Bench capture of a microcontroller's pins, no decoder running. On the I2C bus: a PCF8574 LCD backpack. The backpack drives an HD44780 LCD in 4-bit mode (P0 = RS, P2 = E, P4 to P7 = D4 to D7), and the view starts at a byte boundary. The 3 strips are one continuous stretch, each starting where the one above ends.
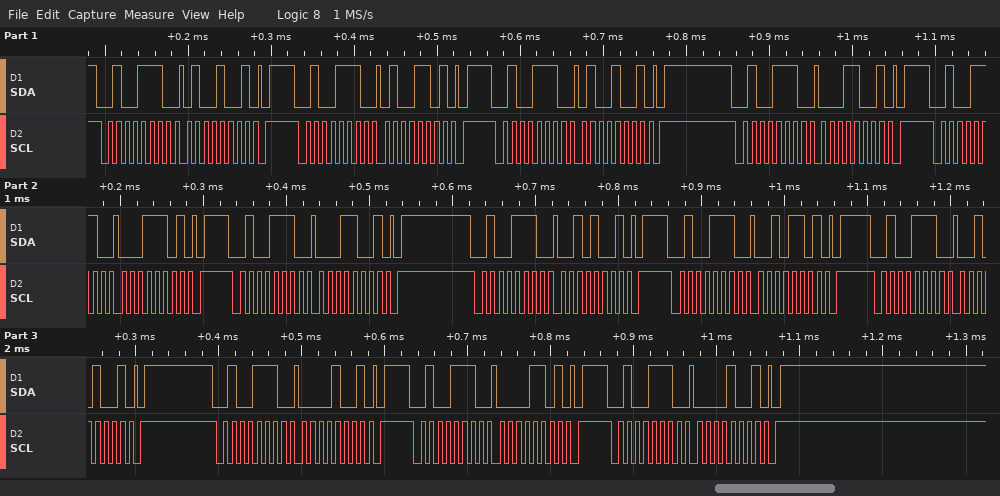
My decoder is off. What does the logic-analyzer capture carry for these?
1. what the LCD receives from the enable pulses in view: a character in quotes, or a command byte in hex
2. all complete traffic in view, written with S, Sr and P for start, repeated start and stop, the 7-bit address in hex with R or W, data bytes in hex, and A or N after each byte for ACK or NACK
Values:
'A' ' '
S 27W A 49 A P S 27W A 4D A P S 27W A 49 A P S 27W A 19 A P S 27W A 1D A P S 27W A 19 A P S 27W A 29 A P S 27W A 2D A P S 27W A 29 A P S 27W A 09 A P S 27W A 0D A P S 27W A 09 A P
